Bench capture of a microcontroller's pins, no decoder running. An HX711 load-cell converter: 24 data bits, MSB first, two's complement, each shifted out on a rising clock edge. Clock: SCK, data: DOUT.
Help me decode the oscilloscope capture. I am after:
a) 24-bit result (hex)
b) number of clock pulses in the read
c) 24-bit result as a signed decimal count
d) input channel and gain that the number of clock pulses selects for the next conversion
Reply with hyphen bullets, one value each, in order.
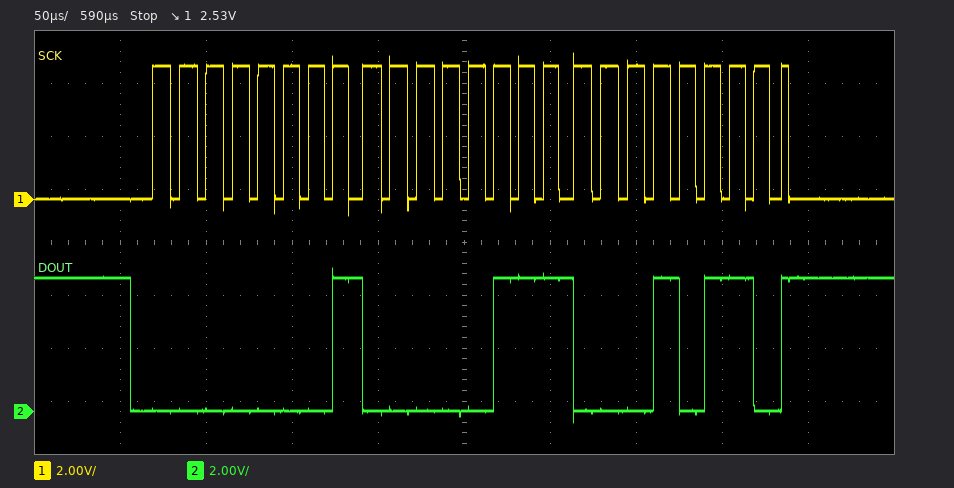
- 0x010716
- 25
- 67350
- channel A, gain 128
